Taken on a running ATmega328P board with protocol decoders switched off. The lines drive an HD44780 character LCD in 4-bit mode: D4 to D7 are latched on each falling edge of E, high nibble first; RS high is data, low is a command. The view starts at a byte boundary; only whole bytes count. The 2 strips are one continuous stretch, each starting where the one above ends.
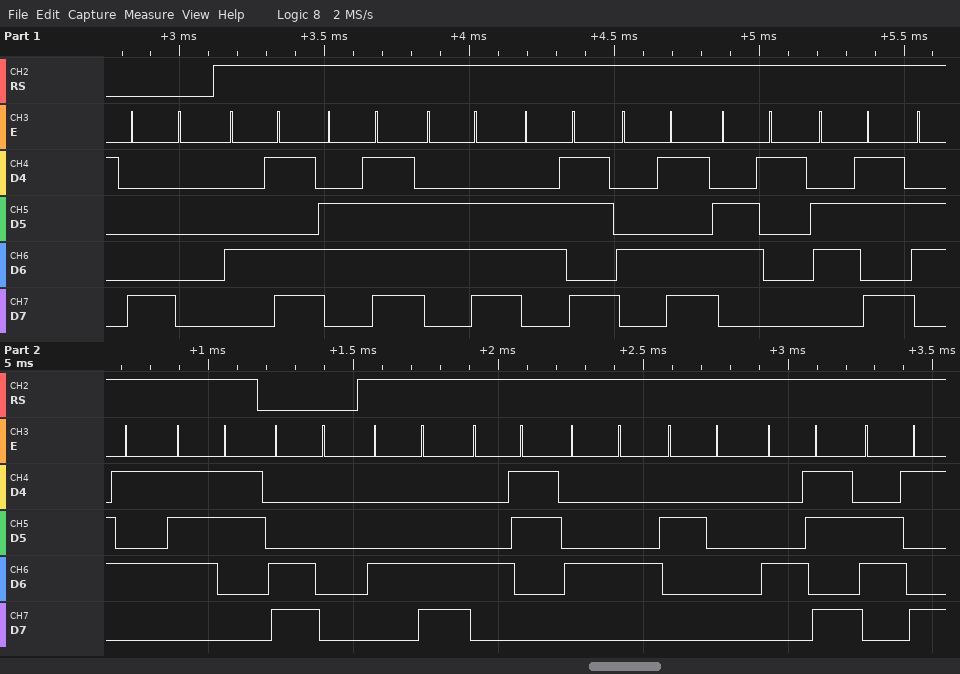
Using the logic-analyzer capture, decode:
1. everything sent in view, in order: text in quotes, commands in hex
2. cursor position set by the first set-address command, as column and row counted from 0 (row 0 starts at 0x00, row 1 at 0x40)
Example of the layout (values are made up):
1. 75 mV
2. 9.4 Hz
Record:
1. 0x80 "MonkMakes" 0xC0 "LCD Ki"
2. column 0, row 0
